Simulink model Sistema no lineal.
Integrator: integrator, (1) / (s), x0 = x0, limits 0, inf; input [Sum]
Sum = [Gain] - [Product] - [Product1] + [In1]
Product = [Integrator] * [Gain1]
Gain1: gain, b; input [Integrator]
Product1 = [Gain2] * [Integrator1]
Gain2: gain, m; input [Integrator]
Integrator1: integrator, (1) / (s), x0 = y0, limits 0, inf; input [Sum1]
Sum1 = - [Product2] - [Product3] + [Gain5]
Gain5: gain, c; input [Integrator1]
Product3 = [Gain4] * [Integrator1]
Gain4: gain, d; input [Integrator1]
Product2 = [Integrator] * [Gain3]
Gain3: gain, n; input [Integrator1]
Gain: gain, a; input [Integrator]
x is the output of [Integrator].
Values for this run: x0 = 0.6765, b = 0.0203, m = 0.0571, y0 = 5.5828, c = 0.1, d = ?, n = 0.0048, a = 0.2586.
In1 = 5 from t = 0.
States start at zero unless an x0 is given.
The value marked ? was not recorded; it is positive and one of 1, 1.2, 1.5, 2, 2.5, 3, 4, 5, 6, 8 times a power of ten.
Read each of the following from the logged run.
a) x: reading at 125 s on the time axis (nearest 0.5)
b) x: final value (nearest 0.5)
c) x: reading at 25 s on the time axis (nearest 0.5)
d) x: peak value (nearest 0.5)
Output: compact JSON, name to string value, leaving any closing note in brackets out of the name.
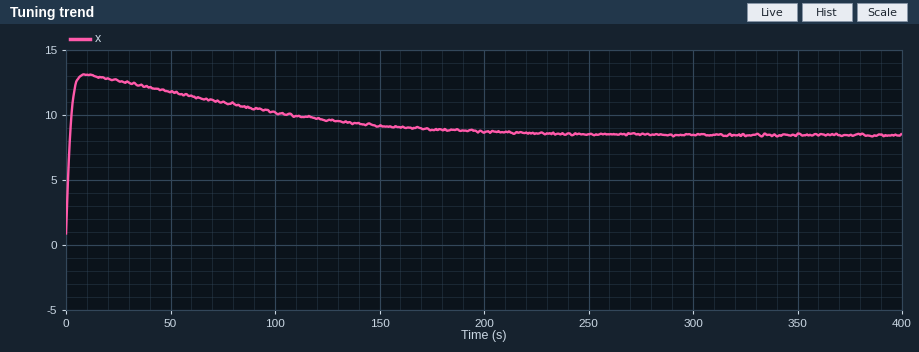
{"x: reading at 125 s on the time axis": "9.5", "x: final value": "8.5", "x: reading at 25 s on the time axis": "12.5", "x: peak value": "13.0"}
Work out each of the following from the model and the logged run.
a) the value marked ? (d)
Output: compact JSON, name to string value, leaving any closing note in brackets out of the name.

{"the value marked ?": "0.005"}
